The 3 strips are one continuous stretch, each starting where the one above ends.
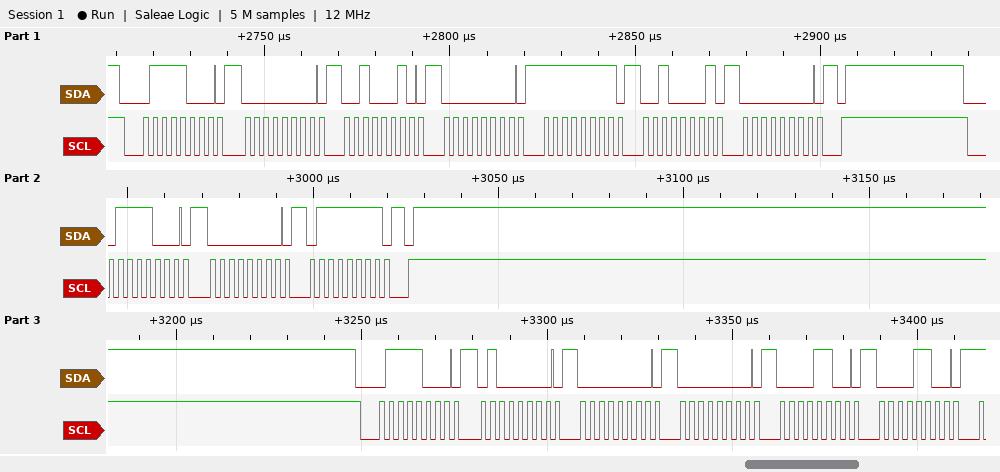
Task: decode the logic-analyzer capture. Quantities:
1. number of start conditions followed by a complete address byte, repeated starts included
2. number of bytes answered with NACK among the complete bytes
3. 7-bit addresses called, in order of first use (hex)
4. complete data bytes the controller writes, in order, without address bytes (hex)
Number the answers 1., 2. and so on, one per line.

1. 3
2. 0
3. 0x3C
4. 00 22 00 FF 21 00 00 7F 40 00 00 0C 0C
